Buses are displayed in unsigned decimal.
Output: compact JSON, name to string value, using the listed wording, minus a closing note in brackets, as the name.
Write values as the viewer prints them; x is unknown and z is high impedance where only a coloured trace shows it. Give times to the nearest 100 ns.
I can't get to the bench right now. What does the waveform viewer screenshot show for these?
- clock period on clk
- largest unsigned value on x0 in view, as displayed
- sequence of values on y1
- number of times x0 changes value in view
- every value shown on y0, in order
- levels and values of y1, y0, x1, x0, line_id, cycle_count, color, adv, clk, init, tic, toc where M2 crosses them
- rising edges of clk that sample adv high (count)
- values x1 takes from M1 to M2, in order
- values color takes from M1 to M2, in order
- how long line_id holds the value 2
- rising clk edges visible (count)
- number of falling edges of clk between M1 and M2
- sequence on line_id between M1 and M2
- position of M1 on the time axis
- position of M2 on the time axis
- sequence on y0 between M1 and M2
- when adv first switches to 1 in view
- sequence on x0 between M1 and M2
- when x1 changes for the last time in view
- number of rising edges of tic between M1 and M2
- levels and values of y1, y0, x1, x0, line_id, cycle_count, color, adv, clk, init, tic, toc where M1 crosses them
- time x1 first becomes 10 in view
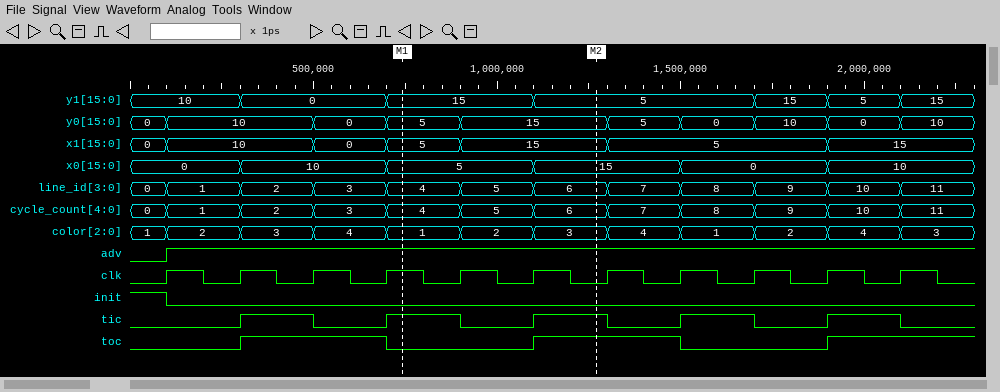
{"clock period on clk": "200 ns", "largest unsigned value on x0 in view, as displayed": "15", "sequence of values on y1": "10, 0, 15, 5, 15, 5, 15", "number of times x0 changes value in view": "5", "every value shown on y0, in order": "0, 10, 0, 5, 15, 5, 0, 10, 0, 10", "levels and values of y1, y0, x1, x0, line_id, cycle_count, color, adv, clk, init, tic, toc where M2 crosses them": "y1=5, y0=15, x1=15, x0=15, line_id=6, cycle_count=6, color=3, adv=1, clk=0, init=0, tic=1, toc=1", "rising edges of clk that sample adv high": "10", "values x1 takes from M1 to M2, in order": "5, 15", "values color takes from M1 to M2, in order": "1, 2, 3", "how long line_id holds the value 2": "200 ns", "rising clk edges visible": "11", "number of falling edges of clk between M1 and M2": "3", "sequence on line_id between M1 and M2": "4, 5, 6", "position of M1 on the time axis": "700 ns", "position of M2 on the time axis": "1300 ns", "sequence on y0 between M1 and M2": "5, 15", "when adv first switches to 1 in view": "100 ns", "sequence on x0 between M1 and M2": "5, 15", "when x1 changes for the last time in view": "1900 ns", "number of rising edges of tic between M1 and M2": "1", "levels and values of y1, y0, x1, x0, line_id, cycle_count, color, adv, clk, init, tic, toc where M1 crosses them": "y1=15, y0=5, x1=5, x0=5, line_id=4, cycle_count=4, color=1, adv=1, clk=1, init=0, tic=1, toc=0", "time x1 first becomes 10 in view": "100 ns"}
